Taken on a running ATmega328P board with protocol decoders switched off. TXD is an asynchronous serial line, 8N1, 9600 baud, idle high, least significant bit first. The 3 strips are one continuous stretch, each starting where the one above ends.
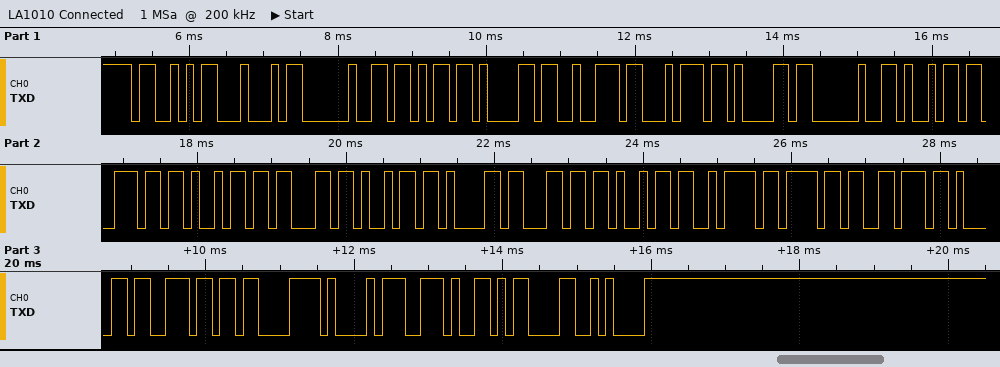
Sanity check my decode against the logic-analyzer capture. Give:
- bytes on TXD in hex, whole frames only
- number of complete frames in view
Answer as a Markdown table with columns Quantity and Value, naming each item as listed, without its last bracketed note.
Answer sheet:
| Quantity | Value |
|---|---|
| bytes on TXD in hex, whole frames only | 0x53 0x44 0x20 0x6B 0x61 0x72 0x74 0x61 0x20 0x69 0x6E 0x69 0x63 0x69 0x61 0x6C 0x69 0x7A 0x6F 0x76 0x61 0x6E 0xC3 0xA1 0x2E 0x0D 0x0A |
| number of complete frames in view | 27 |
